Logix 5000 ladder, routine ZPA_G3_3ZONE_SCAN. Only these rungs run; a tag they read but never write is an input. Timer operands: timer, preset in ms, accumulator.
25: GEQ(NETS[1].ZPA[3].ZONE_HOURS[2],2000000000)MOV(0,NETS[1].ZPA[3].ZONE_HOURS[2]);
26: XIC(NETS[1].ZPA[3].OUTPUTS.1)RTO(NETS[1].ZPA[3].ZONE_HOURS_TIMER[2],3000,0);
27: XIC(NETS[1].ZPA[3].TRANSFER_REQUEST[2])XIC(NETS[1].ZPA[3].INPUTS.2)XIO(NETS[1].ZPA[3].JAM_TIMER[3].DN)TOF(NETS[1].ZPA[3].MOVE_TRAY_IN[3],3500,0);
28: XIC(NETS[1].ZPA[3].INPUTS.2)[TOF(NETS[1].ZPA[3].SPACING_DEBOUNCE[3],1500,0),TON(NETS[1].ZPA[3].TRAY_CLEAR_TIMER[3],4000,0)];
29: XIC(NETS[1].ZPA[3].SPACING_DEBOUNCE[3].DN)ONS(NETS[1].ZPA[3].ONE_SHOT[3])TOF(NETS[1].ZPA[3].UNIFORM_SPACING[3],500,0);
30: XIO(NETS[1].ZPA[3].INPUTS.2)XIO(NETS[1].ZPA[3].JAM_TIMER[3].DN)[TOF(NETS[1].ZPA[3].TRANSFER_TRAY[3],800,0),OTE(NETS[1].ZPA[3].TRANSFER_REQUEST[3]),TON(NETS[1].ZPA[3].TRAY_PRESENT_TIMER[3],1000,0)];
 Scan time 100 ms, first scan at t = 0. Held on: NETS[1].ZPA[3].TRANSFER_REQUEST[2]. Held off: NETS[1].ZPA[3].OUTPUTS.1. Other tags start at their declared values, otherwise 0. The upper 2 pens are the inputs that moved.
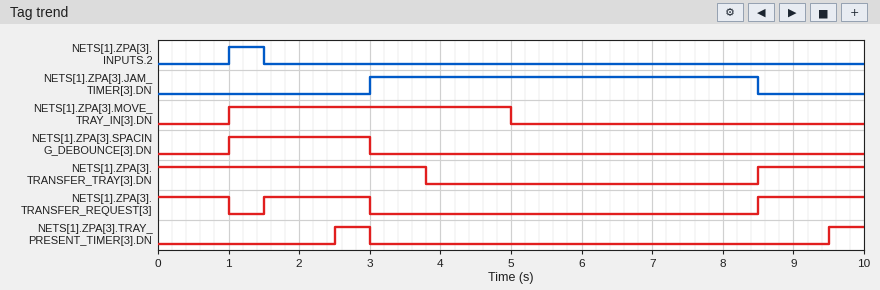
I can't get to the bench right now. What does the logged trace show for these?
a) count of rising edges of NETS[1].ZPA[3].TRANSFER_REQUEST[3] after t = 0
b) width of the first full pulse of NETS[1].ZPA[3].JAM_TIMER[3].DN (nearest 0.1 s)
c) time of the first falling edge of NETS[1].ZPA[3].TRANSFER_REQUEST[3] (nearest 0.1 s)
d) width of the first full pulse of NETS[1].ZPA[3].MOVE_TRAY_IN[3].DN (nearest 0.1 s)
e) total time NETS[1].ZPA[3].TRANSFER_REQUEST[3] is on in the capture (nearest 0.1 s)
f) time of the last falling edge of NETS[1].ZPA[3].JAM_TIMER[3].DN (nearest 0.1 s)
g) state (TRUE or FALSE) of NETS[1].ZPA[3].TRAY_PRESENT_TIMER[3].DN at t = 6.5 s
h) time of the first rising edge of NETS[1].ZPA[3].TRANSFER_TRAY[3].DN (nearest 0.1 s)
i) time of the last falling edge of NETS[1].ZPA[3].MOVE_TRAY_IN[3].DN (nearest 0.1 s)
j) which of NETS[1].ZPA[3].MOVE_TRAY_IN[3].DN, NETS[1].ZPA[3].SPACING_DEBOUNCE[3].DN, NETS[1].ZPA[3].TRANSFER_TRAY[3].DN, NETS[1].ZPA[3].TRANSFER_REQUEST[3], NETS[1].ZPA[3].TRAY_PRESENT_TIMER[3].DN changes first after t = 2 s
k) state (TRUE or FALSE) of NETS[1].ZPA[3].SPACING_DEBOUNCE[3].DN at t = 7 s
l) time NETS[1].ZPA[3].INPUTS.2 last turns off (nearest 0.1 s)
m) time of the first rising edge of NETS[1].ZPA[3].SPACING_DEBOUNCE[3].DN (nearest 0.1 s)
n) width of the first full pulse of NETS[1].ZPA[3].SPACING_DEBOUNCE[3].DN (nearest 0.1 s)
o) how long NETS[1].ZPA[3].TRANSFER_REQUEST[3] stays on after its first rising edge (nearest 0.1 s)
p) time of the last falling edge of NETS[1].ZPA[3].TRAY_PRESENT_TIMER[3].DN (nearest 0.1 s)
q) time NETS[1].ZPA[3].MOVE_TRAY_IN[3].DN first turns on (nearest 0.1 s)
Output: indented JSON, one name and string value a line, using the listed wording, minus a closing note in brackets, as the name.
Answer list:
{
  "count of rising edges of NETS[1].ZPA[3].TRANSFER_REQUEST[3] after t = 0": "2",
  "width of the first full pulse of NETS[1].ZPA[3].JAM_TIMER[3].DN": "5.5 s",
  "time of the first falling edge of NETS[1].ZPA[3].TRANSFER_REQUEST[3]": "1.0 s",
  "width of the first full pulse of NETS[1].ZPA[3].MOVE_TRAY_IN[3].DN": "4.0 s",
  "total time NETS[1].ZPA[3].TRANSFER_REQUEST[3] is on in the capture": "4.0 s",
  "time of the last falling edge of NETS[1].ZPA[3].JAM_TIMER[3].DN": "8.5 s",
  "state (TRUE or FALSE) of NETS[1].ZPA[3].TRAY_PRESENT_TIMER[3].DN at t = 6.5 s": "FALSE",
  "time of the first rising edge of NETS[1].ZPA[3].TRANSFER_TRAY[3].DN": "8.5 s",
  "time of the last falling edge of NETS[1].ZPA[3].MOVE_TRAY_IN[3].DN": "5.0 s",
  "which of NETS[1].ZPA[3].MOVE_TRAY_IN[3].DN, NETS[1].ZPA[3].SPACING_DEBOUNCE[3].DN, NETS[1].ZPA[3].TRANSFER_TRAY[3].DN, NETS[1].ZPA[3].TRANSFER_REQUEST[3], NETS[1].ZPA[3].TRAY_PRESENT_TIMER[3].DN changes first after t = 2 s": "NETS[1].ZPA[3].TRAY_PRESENT_TIMER[3].DN",
  "state (TRUE or FALSE) of NETS[1].ZPA[3].SPACING_DEBOUNCE[3].DN at t = 7 s": "FALSE",
  "time NETS[1].ZPA[3].INPUTS.2 last turns off": "1.5 s",
  "time of the first rising edge of NETS[1].ZPA[3].SPACING_DEBOUNCE[3].DN": "1.0 s",
  "width of the first full pulse of NETS[1].ZPA[3].SPACING_DEBOUNCE[3].DN": "2.0 s",
  "how long NETS[1].ZPA[3].TRANSFER_REQUEST[3] stays on after its first rising edge": "1.5 s",
  "time of the last falling edge of NETS[1].ZPA[3].TRAY_PRESENT_TIMER[3].DN": "3.0 s",
  "time NETS[1].ZPA[3].MOVE_TRAY_IN[3].DN first turns on": "1.0 s"
}
